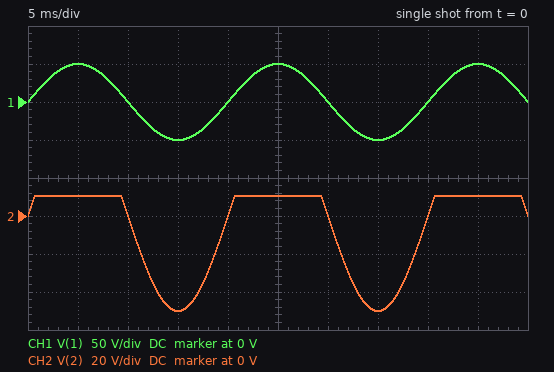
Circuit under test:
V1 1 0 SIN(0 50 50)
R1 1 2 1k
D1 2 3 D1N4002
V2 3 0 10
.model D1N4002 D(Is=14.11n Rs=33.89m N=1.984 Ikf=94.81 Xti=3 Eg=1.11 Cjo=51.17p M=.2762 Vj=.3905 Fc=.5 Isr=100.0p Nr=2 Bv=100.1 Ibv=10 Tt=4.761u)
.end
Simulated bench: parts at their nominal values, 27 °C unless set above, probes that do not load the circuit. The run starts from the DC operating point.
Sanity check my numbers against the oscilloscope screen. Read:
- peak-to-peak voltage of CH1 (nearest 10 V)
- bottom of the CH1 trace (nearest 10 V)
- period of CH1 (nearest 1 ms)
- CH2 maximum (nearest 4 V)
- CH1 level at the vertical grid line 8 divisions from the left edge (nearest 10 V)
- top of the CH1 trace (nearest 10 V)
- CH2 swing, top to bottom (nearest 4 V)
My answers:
100 V
-50 V
20 ms
12 V
0 V
50 V
60 V
